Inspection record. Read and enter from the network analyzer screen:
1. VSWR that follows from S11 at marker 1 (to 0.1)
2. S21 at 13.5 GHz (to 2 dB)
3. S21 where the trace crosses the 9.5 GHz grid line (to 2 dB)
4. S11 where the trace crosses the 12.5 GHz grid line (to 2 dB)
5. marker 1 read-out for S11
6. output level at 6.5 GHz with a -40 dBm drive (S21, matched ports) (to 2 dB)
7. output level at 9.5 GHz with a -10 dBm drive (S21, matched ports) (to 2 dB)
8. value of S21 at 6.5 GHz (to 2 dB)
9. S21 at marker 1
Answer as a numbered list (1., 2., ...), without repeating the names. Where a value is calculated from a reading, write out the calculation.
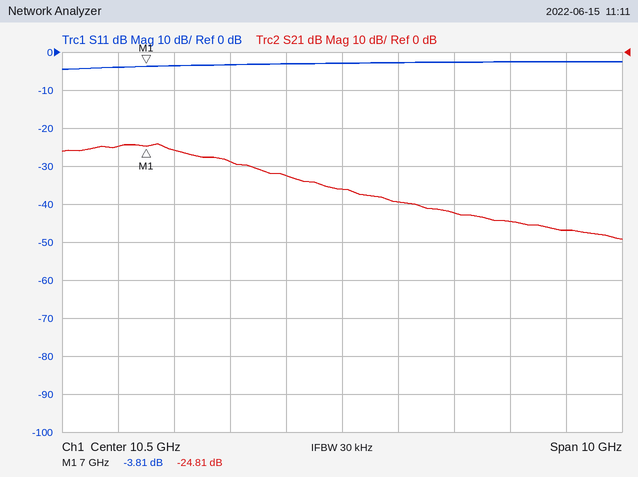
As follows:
1. (1 + 0.6449)/(1 − 0.6449) ≈ 4.6
2. -44 dB
3. -32 dB
4. -2 dB
5. -3.81 dB
6. -40 dBm + (-24 dB) = -64 dBm
7. -10 dBm + (-32 dB) = -42 dBm
8. -24 dB
9. -24.81 dB
